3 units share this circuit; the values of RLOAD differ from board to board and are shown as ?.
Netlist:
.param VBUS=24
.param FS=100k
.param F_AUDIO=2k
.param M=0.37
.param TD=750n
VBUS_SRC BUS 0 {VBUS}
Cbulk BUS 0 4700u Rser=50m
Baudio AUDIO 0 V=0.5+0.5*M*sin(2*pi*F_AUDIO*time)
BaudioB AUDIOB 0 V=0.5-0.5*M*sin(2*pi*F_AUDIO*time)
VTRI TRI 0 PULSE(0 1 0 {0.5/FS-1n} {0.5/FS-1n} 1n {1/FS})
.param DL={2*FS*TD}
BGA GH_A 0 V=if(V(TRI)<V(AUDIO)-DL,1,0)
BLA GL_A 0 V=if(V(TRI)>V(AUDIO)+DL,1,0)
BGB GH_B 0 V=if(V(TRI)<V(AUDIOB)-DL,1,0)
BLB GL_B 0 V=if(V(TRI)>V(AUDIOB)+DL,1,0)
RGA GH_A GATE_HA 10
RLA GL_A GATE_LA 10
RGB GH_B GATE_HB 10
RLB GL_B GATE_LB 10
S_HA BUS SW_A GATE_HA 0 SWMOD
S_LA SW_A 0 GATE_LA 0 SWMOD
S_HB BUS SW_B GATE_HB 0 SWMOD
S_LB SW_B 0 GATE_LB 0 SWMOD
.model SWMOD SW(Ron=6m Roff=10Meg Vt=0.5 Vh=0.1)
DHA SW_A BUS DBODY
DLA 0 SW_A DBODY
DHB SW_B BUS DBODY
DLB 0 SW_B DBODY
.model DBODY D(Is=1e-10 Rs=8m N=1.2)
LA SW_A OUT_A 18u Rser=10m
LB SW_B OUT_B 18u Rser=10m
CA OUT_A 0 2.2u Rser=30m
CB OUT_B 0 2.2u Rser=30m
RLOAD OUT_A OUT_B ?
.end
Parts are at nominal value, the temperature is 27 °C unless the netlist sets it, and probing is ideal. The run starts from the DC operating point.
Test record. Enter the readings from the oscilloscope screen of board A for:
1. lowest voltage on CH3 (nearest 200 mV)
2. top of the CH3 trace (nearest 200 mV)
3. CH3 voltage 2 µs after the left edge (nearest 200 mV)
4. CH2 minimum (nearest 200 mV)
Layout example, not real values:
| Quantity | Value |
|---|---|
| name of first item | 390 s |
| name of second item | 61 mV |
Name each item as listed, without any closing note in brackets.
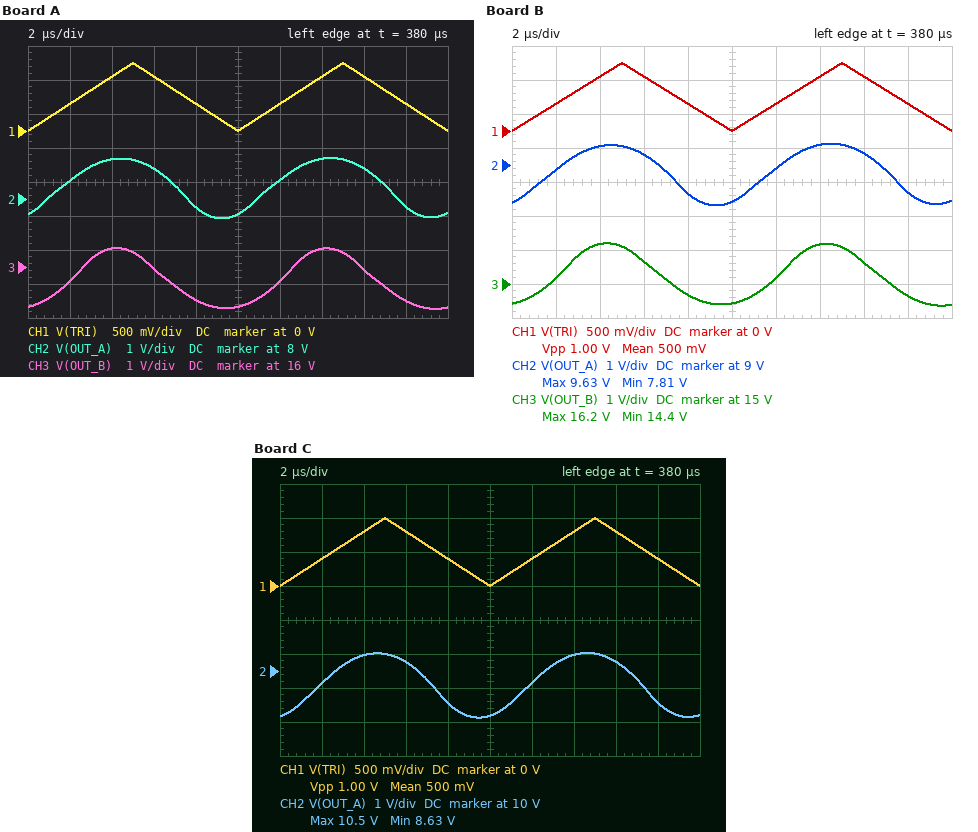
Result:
| Quantity | Value |
|---|---|
| lowest voltage on CH3 | 14.8 V |
| top of the CH3 trace | 16.6 V |
| CH3 voltage 2 µs after the left edge | 15.6 V |
| CH2 minimum | 7.4 V |
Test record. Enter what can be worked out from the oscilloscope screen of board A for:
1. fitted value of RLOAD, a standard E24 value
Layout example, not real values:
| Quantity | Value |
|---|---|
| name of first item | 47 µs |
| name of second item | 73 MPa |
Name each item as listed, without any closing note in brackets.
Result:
| Quantity | Value |
|---|---|
| fitted value of RLOAD, a standard E24 value | 6.8 Ω |
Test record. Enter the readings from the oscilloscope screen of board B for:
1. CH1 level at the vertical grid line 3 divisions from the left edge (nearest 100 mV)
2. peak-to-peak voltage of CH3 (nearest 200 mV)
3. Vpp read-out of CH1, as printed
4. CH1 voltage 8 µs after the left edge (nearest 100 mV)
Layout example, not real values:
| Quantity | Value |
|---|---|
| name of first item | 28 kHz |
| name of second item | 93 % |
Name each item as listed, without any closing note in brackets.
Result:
| Quantity | Value |
|---|---|
| CH1 level at the vertical grid line 3 divisions from the left edge | 800 mV |
| peak-to-peak voltage of CH3 | 1.8 V |
| Vpp read-out of CH1, as printed | 1.00 V |
| CH1 voltage 8 µs after the left edge | 400 mV |
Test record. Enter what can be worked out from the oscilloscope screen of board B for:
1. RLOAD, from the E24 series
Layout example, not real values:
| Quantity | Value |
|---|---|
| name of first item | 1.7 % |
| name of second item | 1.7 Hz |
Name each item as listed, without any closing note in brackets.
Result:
| Quantity | Value |
|---|---|
| RLOAD, from the E24 series | 5.6 Ω |
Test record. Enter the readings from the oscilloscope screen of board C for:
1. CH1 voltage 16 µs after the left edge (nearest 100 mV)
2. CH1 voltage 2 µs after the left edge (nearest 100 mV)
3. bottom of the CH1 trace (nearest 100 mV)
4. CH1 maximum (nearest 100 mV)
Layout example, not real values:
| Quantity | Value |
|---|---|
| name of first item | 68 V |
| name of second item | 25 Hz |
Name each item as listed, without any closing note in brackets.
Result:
| Quantity | Value |
|---|---|
| CH1 voltage 16 µs after the left edge | 800 mV |
| CH1 voltage 2 µs after the left edge | 400 mV |
| bottom of the CH1 trace | 0 V |
| CH1 maximum | 1.0 V |
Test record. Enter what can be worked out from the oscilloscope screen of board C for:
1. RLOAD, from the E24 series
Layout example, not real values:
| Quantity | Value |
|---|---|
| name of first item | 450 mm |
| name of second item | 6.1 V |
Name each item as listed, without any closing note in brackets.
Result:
| Quantity | Value |
|---|---|
| RLOAD, from the E24 series | 3.6 Ω |
